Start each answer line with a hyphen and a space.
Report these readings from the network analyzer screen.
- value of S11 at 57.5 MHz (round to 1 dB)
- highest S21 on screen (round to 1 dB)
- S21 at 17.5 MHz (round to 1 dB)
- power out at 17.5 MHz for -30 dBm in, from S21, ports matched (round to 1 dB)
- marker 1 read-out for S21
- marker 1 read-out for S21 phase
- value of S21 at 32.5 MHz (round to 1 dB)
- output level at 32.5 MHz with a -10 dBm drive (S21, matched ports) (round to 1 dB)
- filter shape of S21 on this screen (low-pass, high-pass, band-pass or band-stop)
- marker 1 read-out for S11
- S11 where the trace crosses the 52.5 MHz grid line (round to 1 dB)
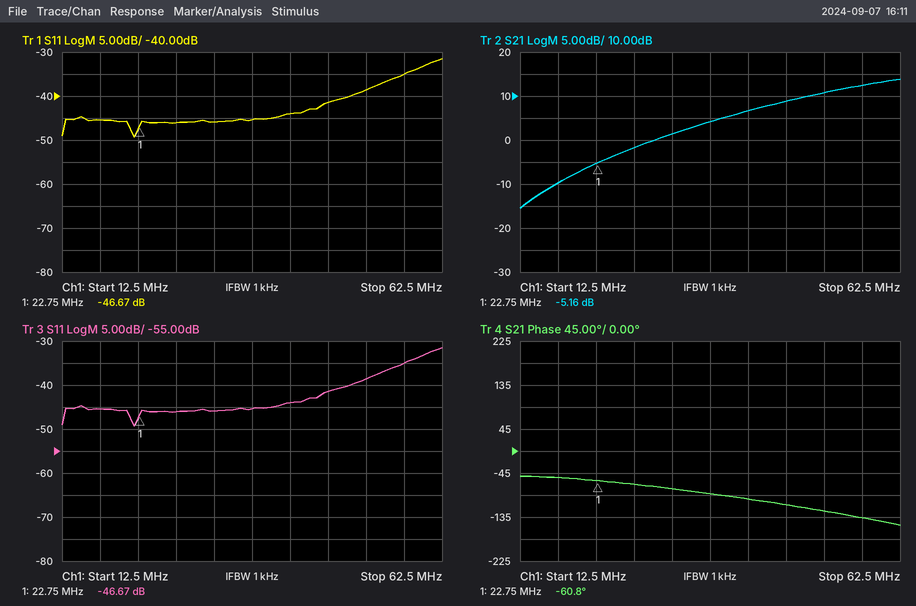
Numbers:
- -35 dB
- 14 dB
- -10 dB
- -40 dBm
- -5.16 dB
- -60.8°
- 1 dB
- -9 dBm
- high-pass
- -46.67 dB
- -39 dB
